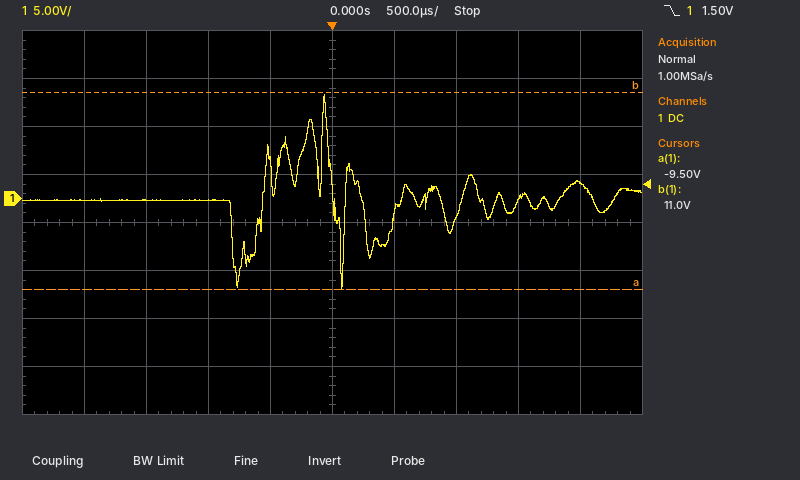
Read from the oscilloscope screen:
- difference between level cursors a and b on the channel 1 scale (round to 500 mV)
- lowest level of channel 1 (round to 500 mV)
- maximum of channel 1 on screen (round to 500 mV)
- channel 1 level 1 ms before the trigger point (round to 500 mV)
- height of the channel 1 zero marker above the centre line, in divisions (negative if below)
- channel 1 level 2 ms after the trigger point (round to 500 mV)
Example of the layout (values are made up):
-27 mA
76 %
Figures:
20.5 V
-9.5 V
11.0 V
0.0 V
+0.5 div
1.5 V
